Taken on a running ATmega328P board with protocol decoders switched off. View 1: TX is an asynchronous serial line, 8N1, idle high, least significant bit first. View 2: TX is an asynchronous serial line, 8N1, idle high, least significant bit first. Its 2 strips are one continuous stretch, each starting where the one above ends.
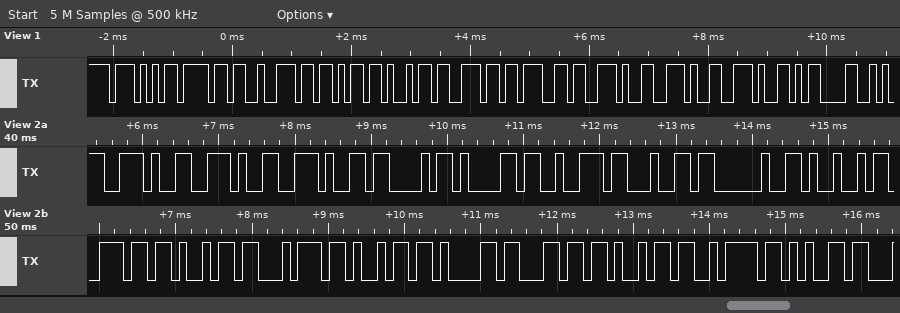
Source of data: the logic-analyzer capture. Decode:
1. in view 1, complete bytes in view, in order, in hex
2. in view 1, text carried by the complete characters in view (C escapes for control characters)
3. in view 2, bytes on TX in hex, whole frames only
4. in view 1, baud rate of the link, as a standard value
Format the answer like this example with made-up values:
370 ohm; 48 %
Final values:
57 6F 72 6B 69 6E 67 2E 2E 2E 0D; "Working...\r"; 2E 2E 2E 43 61 72 64 20 49 6E 69 74 69 61 6C 69 7A 65; 9600 baud
